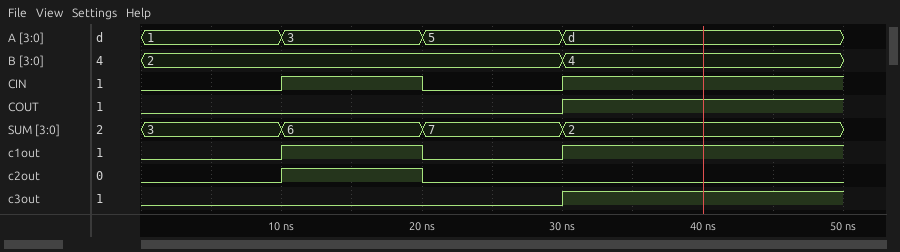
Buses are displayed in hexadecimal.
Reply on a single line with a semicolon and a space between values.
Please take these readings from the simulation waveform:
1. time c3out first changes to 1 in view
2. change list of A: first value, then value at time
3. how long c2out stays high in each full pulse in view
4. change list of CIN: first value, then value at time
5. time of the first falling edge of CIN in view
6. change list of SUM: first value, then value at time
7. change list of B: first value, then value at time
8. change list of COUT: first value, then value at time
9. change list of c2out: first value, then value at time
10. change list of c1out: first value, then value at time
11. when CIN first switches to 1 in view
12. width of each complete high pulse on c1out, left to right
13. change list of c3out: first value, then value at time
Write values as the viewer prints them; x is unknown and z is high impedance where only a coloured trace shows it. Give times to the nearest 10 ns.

30 ns; 1, 3 at 10 ns, 5 at 20 ns, d at 30 ns; 10 ns; 0, 1 at 10 ns, 0 at 20 ns, 1 at 30 ns; 20 ns; 3, 6 at 10 ns, 7 at 20 ns, 2 at 30 ns; 2, 4 at 30 ns; 0, 1 at 30 ns; 0, 1 at 10 ns, 0 at 20 ns; 0, 1 at 10 ns, 0 at 20 ns, 1 at 30 ns; 10 ns; 10 ns; 0, 1 at 30 ns
